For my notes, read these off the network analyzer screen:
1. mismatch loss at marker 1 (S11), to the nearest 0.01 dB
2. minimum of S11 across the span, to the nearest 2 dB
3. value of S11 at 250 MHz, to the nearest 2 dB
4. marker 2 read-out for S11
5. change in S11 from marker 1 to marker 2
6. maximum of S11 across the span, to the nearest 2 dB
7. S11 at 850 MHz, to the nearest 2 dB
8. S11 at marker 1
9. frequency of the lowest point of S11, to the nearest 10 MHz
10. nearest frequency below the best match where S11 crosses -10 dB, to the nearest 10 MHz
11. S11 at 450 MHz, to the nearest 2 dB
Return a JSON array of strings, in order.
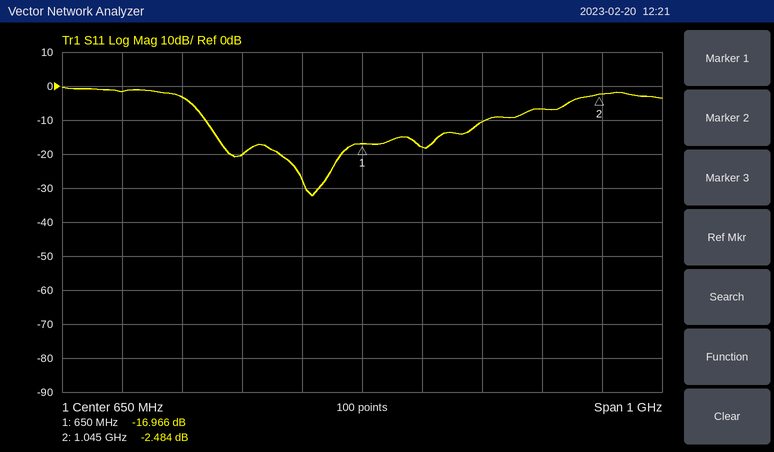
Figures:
["0.09 dB", "-32 dB", "-2 dB", "-2.484 dB", "14.482 dB", "0 dB", "-10 dB", "-16.966 dB", "570 MHz", "390 MHz", "-20 dB"]
